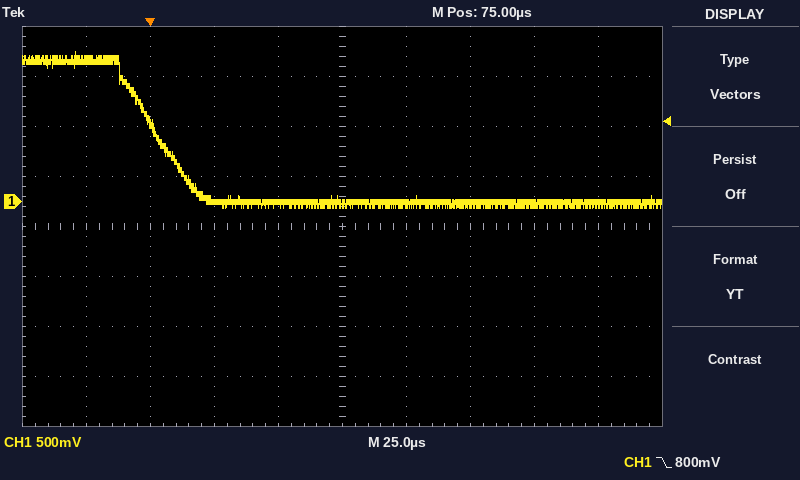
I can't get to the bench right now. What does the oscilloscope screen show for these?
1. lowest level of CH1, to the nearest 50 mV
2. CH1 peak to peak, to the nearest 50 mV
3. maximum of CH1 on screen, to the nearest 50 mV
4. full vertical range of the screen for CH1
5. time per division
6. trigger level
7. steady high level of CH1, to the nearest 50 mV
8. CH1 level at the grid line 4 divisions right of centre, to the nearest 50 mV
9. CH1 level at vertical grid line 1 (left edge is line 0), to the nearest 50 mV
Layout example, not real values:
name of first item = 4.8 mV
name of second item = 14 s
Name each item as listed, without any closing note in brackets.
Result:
lowest level of CH1, to the nearest 50 mV = -50 mV
CH1 peak to peak, to the nearest 50 mV = 1.55 V
maximum of CH1 on screen, to the nearest 50 mV = 1.50 V
full vertical range of the screen for CH1 = 4 V
time per division = 25 µs
trigger level = 800 mV
steady high level of CH1, to the nearest 50 mV = 1.40 V
CH1 level at the grid line 4 divisions right of centre, to the nearest 50 mV = 0 mV
CH1 level at vertical grid line 1 (left edge is line 0), to the nearest 50 mV = 1.40 V
